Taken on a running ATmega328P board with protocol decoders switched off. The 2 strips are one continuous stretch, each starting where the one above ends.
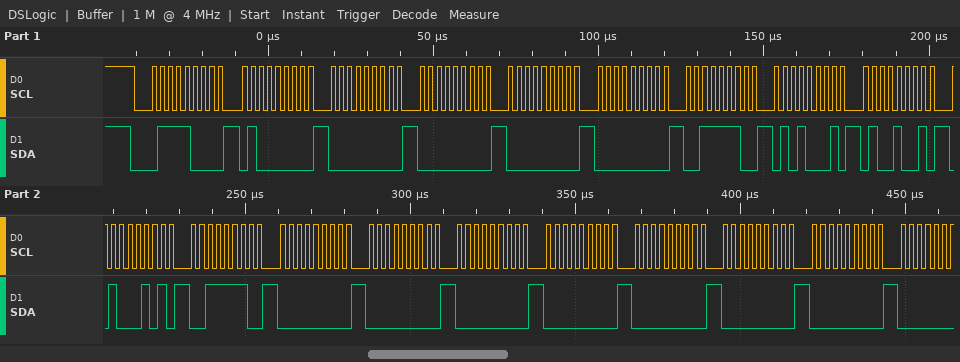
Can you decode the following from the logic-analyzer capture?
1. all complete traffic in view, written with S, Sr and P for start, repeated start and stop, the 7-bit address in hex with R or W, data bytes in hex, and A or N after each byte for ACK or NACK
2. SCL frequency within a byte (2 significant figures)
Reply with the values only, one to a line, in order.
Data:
S 3CW A 40 A 00 A 00 A 00 A 00 A 3E A 51 A 49 A 45 A 3E A 00 A 00 A 00 A 00 A 00 A 00 A 00 A
400 kHz
